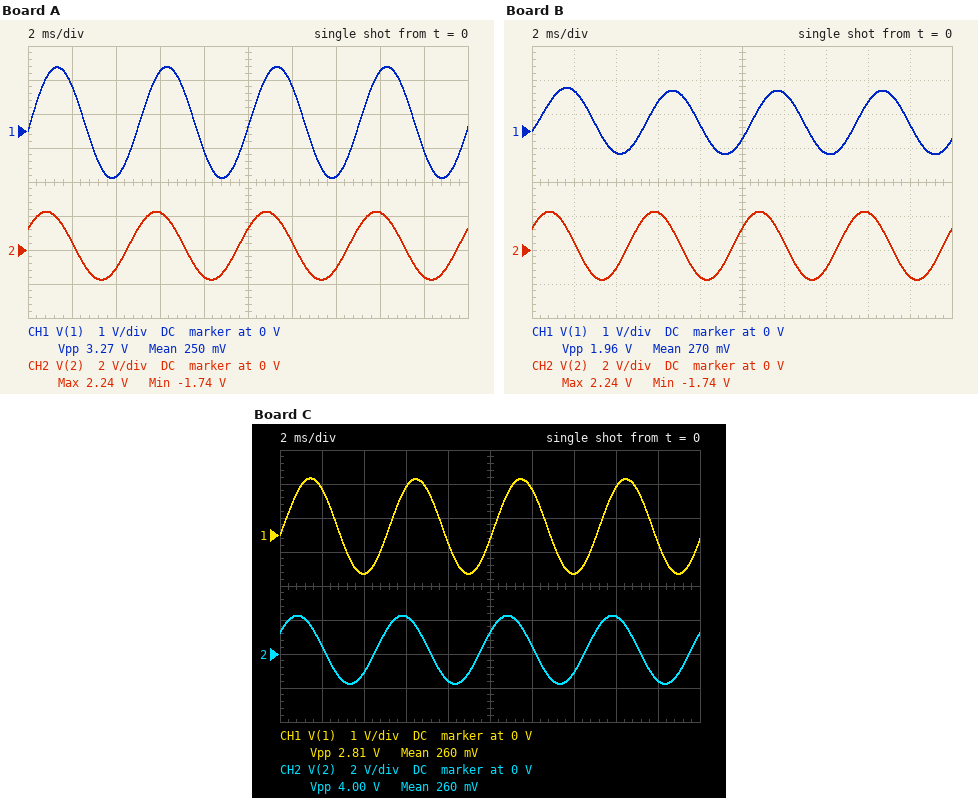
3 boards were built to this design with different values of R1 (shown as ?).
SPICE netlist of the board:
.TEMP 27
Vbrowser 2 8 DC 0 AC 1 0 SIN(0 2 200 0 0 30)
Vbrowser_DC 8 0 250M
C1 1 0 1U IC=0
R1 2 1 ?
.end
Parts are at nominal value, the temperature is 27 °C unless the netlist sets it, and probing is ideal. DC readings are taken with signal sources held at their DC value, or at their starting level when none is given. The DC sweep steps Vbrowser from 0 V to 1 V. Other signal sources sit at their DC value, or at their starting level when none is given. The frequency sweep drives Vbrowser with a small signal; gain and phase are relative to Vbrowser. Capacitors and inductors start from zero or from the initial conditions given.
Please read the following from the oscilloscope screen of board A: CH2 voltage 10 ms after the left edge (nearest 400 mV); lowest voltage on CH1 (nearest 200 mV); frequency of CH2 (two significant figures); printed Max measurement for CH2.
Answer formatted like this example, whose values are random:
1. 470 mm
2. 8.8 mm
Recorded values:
1. 1.2 V
2. -1.4 V
3. 200 Hz
4. 2.24 V
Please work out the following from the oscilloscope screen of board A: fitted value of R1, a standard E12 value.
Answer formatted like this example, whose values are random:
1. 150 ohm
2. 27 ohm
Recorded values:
1. 560 Ω
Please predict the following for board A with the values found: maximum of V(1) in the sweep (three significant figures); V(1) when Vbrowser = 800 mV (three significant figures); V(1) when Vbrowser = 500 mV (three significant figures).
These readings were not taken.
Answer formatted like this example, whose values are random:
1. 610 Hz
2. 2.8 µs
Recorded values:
1. 1.25 V
2. 1.05 V
3. 750 mV
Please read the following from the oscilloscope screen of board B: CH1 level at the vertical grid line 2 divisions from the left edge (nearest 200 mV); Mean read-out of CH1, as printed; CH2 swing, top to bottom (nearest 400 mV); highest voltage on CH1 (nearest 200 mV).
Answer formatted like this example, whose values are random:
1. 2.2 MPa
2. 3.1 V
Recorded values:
1. -600 mV
2. 270 mV
3. 4.0 V
4. 1.2 V
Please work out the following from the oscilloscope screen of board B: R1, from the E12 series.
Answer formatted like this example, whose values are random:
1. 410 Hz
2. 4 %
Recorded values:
1. 1.5 kΩ
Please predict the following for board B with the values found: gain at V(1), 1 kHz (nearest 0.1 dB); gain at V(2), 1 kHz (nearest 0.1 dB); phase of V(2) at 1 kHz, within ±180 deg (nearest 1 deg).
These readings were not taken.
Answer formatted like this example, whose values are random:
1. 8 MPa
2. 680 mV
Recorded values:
1. -19.5 dB
2. 0 dB
3. 0 deg
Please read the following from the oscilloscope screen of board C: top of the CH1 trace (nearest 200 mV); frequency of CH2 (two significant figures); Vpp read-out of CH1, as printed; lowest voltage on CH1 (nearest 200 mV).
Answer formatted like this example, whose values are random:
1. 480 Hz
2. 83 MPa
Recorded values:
1. 1.6 V
2. 200 Hz
3. 2.81 V
4. -1.2 V
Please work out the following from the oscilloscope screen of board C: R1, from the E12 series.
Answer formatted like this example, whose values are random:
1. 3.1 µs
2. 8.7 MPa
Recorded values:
1. 820 Ω
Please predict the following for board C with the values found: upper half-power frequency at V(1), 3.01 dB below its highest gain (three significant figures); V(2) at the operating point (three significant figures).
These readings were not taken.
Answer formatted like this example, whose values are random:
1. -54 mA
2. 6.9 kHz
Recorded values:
1. 194 Hz
2. 250 mV
